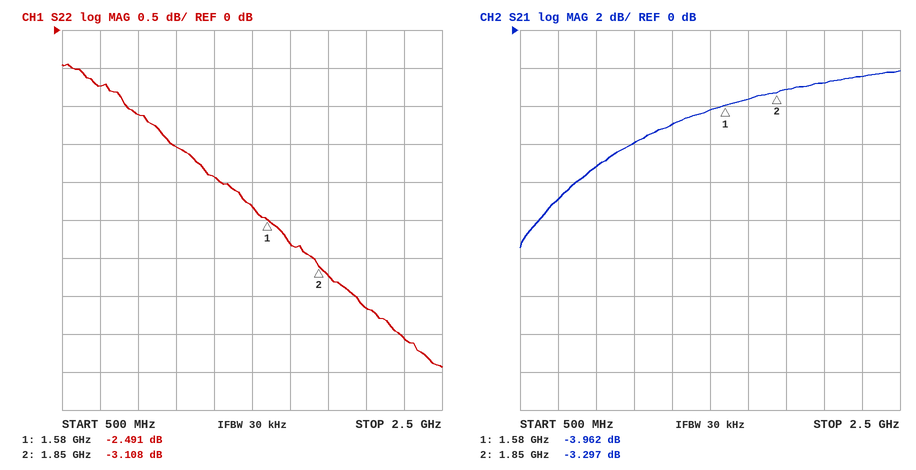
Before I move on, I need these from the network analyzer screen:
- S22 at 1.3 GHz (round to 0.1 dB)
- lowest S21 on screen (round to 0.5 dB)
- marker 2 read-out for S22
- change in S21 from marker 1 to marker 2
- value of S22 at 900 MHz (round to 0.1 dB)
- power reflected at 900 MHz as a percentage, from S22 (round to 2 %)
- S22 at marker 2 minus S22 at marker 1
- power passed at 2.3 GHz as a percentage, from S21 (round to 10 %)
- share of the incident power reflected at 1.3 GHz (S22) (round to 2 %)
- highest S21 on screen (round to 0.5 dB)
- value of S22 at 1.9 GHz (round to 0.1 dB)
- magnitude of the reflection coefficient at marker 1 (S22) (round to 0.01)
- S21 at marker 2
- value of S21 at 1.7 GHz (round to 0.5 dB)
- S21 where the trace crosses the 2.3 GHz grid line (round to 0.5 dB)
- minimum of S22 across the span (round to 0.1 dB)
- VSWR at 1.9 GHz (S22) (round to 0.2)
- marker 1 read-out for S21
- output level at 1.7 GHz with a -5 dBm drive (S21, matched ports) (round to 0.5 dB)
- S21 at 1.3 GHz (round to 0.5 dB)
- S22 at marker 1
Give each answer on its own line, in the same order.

-1.9 dB
-11.5 dB
-3.108 dB
0.665 dB
-1.1 dB
78 %
-0.617 dB
60 %
64 %
-2.0 dB
-3.2 dB
0.75
-3.297 dB
-3.5 dB
-2.5 dB
-4.4 dB
5.4
-3.962 dB
-8.5 dBm
-5.0 dB
-2.491 dB
